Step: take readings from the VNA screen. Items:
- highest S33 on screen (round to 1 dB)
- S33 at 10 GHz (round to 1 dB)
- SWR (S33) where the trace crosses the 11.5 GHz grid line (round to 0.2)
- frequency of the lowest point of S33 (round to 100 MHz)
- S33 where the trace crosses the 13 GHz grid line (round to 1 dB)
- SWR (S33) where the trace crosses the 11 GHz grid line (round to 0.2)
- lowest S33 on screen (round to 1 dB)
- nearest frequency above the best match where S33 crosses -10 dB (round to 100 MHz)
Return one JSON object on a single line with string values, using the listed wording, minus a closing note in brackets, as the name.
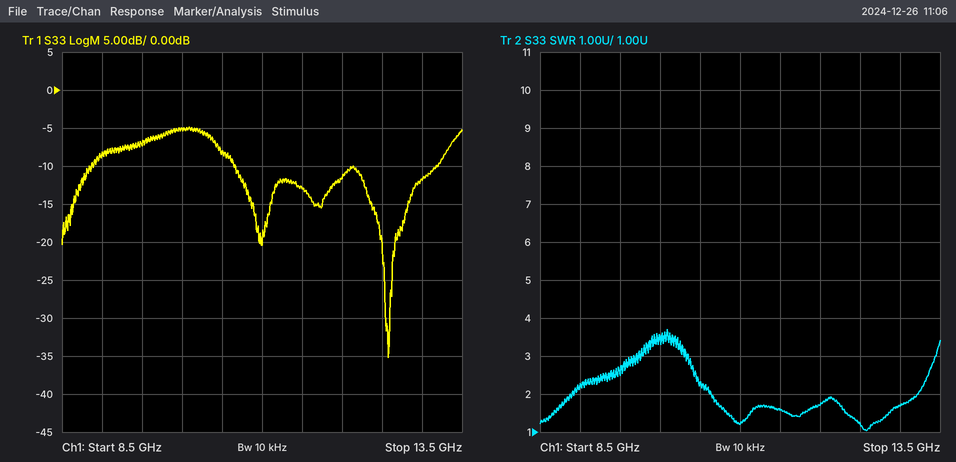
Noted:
{"highest S33 on screen": "-5 dB", "S33 at 10 GHz": "-5 dB", "SWR (S33) where the trace crosses the 11.5 GHz grid line": "1.6", "frequency of the lowest point of S33": "12.6 GHz", "S33 where the trace crosses the 13 GHz grid line": "-12 dB", "SWR (S33) where the trace crosses the 11 GHz grid line": "1.2", "lowest S33 on screen": "-35 dB", "nearest frequency above the best match where S33 crosses -10 dB": "13.2 GHz"}
